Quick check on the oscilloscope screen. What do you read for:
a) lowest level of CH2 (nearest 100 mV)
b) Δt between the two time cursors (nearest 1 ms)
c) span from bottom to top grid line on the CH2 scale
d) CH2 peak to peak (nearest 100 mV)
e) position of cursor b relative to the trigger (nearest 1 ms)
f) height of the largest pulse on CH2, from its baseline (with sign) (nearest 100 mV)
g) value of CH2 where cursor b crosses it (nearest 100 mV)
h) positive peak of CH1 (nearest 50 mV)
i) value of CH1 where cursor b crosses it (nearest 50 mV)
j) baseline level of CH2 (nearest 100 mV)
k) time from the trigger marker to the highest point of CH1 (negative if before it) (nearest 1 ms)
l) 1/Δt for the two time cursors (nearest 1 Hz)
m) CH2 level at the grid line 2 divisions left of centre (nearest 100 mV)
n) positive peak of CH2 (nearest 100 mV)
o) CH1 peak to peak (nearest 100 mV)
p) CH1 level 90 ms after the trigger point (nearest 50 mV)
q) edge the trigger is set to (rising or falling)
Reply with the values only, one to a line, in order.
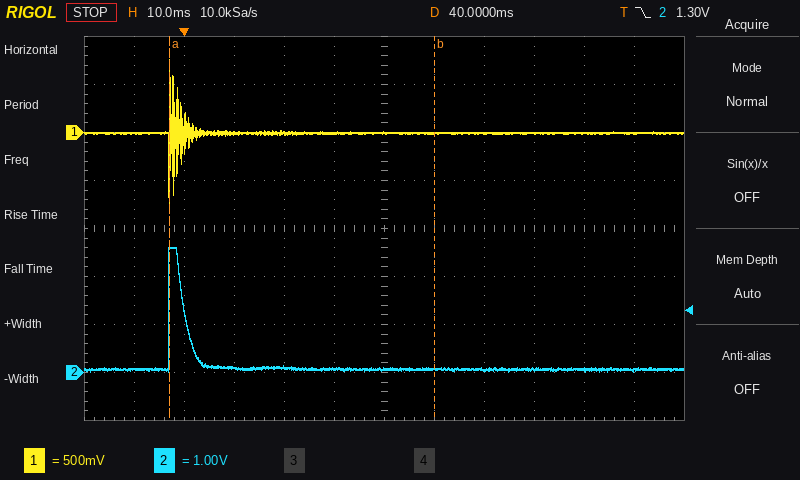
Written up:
0.0 V
53 ms
8 V
2.6 V
+50 ms
+2.5 V
100 mV
750 mV
0 mV
100 mV
-3 ms
19 Hz
100 mV
2.6 V
1.50 V
0 mV
falling
